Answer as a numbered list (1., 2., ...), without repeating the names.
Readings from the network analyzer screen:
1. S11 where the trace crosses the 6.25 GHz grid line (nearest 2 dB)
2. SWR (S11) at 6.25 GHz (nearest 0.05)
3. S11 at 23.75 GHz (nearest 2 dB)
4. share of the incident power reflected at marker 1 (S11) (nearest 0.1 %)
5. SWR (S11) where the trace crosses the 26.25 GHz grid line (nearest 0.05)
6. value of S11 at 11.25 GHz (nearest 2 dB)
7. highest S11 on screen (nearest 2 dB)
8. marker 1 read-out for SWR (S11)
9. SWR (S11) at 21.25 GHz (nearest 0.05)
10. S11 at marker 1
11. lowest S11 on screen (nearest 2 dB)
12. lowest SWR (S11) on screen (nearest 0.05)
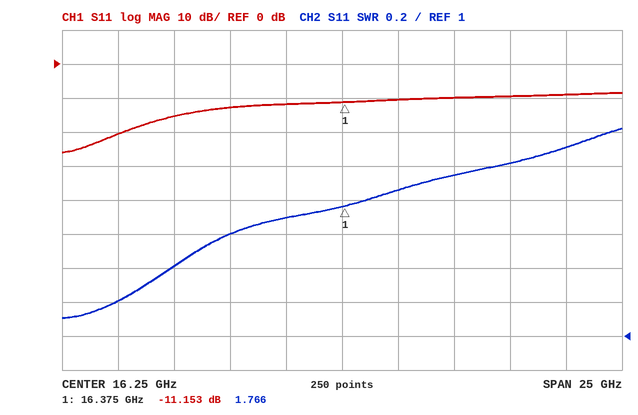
1. -20 dB
2. 1.20
3. -10 dB
4. 7.7 %
5. 2.10
6. -12 dB
7. -8 dB
8. 1.766
9. 1.95
10. -11.153 dB
11. -26 dB
12. 1.10
